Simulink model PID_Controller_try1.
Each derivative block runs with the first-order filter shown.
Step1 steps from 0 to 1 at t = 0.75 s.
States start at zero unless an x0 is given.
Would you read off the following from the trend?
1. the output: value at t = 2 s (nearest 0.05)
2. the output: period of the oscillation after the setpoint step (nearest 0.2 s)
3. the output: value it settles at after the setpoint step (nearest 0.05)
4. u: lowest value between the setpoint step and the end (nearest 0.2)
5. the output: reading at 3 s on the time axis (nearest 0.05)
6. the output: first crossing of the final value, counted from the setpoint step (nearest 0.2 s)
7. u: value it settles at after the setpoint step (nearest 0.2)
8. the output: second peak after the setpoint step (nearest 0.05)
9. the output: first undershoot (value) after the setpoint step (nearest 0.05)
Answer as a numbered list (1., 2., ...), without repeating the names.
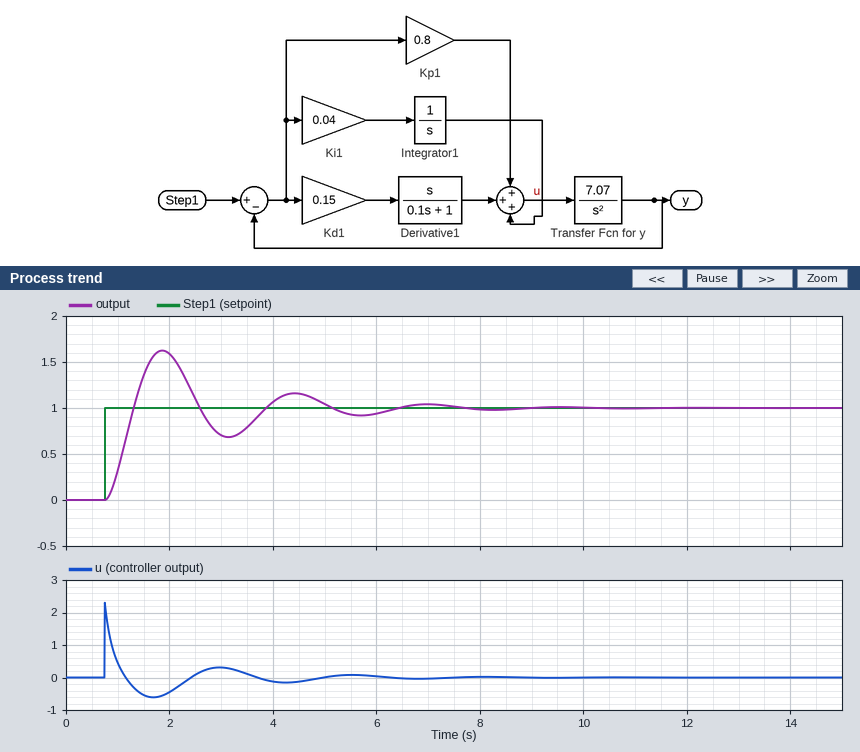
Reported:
1. 1.60
2. 2.6 s
3. 1.00
4. -0.6
5. 0.70
6. 0.6 s
7. 0.0
8. 1.15
9. 0.70
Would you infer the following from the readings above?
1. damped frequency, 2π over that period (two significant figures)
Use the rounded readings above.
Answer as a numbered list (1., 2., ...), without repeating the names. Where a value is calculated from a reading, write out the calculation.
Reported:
1. 2π / 2.6 = 2.4 rad/s
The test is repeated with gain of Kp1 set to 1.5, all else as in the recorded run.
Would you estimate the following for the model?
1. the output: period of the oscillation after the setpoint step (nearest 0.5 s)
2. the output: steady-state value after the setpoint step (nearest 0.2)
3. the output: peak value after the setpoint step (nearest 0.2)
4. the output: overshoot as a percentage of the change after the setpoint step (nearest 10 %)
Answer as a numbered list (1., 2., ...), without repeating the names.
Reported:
1. 2.0 s
2. 1.0
3. 1.8
4. 70 %
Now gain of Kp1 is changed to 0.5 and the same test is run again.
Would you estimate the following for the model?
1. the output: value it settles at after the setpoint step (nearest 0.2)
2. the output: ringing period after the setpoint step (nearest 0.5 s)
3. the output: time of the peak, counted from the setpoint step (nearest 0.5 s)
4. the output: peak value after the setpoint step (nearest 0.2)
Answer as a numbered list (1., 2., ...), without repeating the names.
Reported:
1. 1.0
2. 3.5 s
3. 1.5 s
4. 1.6
